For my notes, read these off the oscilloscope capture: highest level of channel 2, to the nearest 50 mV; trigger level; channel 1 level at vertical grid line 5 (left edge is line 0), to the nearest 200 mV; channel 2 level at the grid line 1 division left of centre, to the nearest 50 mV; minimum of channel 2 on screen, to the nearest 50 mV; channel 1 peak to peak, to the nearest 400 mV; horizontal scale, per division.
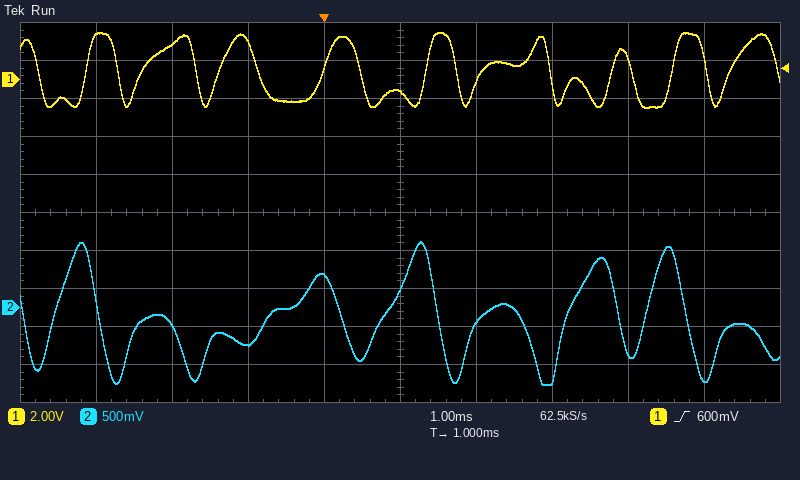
850 mV
600 mV
-600 mV
400 mV
-1.00 V
4.0 V
1 ms
